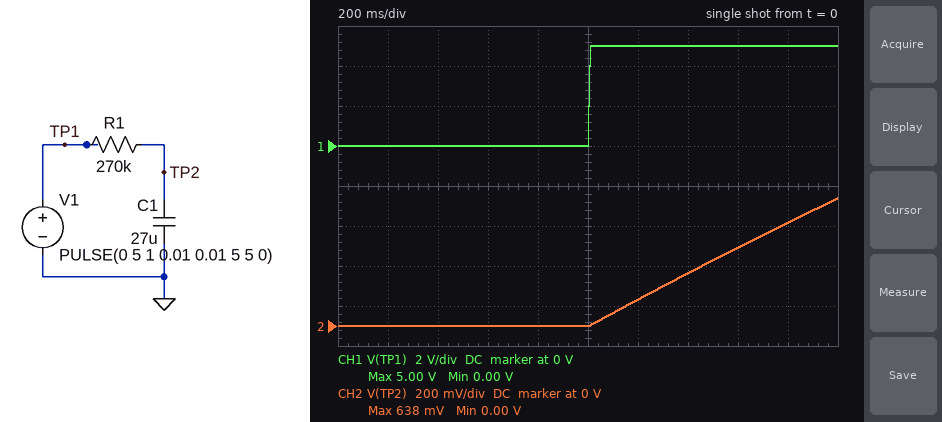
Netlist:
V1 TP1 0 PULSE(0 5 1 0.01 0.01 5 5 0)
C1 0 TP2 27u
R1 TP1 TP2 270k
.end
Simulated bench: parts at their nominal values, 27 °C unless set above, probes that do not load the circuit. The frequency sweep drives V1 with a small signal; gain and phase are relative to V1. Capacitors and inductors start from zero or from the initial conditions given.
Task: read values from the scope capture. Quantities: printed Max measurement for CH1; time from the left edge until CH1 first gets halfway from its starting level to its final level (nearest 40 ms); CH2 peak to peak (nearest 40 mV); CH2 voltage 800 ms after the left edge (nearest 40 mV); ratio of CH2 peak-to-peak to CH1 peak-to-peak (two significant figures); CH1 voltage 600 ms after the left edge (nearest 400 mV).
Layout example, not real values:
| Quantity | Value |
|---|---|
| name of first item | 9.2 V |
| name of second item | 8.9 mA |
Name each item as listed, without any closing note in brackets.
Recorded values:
| Quantity | Value |
|---|---|
| printed Max measurement for CH1 | 5.00 V |
| time from the left edge until CH1 first gets halfway from its starting level to its final level | 1.00 s |
| CH2 peak to peak | 640 mV |
| CH2 voltage 800 ms after the left edge | 0 V |
| ratio of CH2 peak-to-peak to CH1 peak-to-peak | 0.13 |
| CH1 voltage 600 ms after the left edge | 0 V |
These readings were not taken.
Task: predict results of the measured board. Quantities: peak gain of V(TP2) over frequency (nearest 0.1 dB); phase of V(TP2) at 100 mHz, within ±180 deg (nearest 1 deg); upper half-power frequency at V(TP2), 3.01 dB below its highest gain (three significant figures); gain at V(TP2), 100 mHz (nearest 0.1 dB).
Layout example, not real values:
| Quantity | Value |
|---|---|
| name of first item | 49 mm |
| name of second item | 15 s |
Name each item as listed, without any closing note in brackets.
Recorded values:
| Quantity | Value |
|---|---|
| peak gain of V(TP2) over frequency | 0 dB |
| phase of V(TP2) at 100 mHz, within ±180 deg | -78 deg |
| upper half-power frequency at V(TP2), 3.01 dB below its highest gain | 21.8 mHz |
| gain at V(TP2), 100 mHz | -13.4 dB |
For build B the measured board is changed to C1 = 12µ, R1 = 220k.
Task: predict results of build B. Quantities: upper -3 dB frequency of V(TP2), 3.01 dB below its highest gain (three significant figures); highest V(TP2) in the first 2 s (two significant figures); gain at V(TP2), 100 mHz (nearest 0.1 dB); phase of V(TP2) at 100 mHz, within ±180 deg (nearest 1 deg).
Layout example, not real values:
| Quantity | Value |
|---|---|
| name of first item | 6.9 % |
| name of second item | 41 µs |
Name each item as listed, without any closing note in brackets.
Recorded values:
| Quantity | Value |
|---|---|
| upper -3 dB frequency of V(TP2), 3.01 dB below its highest gain | 60.3 mHz |
| highest V(TP2) in the first 2 s | 1.6 V |
| gain at V(TP2), 100 mHz | -5.7 dB |
| phase of V(TP2) at 100 mHz, within ±180 deg | -59 deg |
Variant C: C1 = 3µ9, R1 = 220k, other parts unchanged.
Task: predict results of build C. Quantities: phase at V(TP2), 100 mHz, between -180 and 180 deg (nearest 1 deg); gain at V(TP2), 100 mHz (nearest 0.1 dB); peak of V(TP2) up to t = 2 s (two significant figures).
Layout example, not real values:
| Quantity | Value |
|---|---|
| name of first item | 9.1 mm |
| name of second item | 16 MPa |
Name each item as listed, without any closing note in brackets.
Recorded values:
| Quantity | Value |
|---|---|
| phase at V(TP2), 100 mHz, between -180 and 180 deg | -28 deg |
| gain at V(TP2), 100 mHz | -1.1 dB |
| peak of V(TP2) up to t = 2 s | 3.4 V |
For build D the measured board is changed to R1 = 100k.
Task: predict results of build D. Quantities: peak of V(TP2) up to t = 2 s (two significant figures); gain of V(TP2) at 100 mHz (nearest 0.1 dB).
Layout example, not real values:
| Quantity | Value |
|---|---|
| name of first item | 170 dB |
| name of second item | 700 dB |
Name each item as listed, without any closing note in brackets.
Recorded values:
| Quantity | Value |
|---|---|
| peak of V(TP2) up to t = 2 s | 1.5 V |
| gain of V(TP2) at 100 mHz | -5.9 dB |
